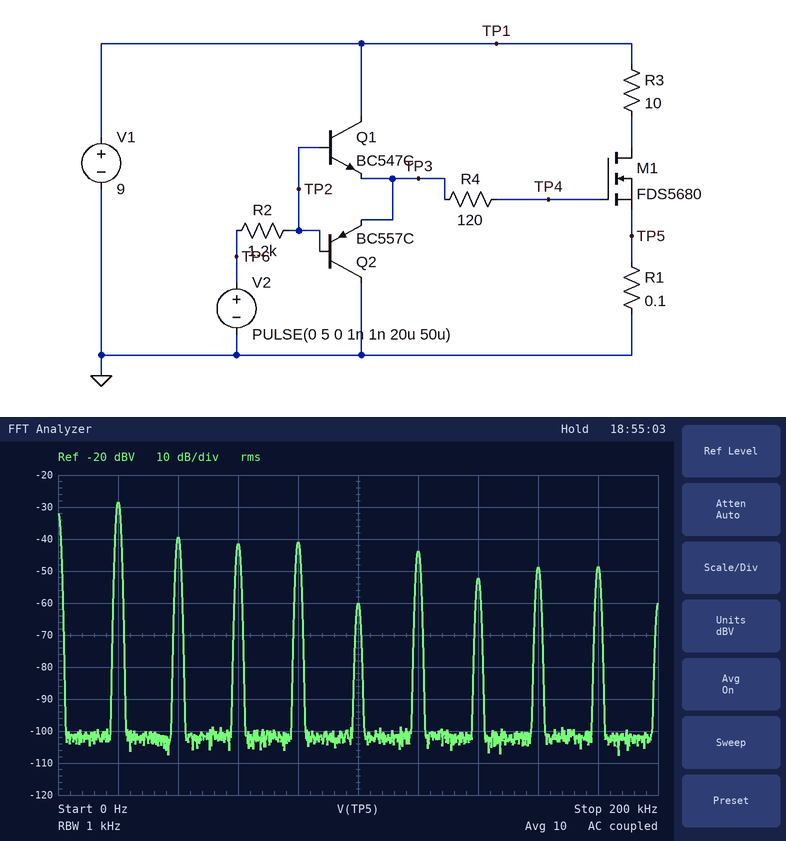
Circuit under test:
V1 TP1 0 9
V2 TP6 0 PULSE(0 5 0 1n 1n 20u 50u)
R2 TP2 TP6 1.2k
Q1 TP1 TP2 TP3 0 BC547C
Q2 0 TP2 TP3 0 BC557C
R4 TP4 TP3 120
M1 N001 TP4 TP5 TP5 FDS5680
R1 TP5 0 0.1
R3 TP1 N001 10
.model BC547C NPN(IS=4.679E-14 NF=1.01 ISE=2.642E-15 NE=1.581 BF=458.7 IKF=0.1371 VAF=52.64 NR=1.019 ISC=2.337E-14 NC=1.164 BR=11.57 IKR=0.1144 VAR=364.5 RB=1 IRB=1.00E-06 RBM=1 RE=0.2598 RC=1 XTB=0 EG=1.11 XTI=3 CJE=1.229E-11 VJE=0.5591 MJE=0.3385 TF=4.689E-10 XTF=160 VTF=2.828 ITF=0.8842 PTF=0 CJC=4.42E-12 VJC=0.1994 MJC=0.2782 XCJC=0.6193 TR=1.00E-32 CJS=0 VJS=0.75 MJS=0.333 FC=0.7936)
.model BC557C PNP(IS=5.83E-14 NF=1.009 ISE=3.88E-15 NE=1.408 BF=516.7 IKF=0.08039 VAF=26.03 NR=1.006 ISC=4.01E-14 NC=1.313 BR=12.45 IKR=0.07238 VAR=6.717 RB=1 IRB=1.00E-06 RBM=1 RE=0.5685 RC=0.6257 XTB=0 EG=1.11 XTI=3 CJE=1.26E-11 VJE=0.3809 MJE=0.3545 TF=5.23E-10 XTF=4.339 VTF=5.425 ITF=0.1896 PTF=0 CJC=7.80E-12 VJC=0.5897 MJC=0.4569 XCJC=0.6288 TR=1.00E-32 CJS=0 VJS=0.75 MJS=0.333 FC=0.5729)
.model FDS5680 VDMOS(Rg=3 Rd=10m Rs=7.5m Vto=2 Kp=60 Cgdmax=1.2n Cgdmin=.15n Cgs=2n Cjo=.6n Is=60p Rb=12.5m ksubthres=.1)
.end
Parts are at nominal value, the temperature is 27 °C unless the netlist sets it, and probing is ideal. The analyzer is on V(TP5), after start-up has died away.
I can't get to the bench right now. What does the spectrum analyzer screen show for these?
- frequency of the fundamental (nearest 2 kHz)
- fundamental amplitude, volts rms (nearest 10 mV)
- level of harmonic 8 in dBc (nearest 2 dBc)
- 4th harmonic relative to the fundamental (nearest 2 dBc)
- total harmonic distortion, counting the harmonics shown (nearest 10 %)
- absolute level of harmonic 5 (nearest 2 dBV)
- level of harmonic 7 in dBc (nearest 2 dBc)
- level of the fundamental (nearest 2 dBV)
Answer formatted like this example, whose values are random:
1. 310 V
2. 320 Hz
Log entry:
1. 20 kHz
2. 40 mV
3. -20 dBc
4. -12 dBc
5. 50 %
6. -60 dBV
7. -24 dBc
8. -28 dBV
